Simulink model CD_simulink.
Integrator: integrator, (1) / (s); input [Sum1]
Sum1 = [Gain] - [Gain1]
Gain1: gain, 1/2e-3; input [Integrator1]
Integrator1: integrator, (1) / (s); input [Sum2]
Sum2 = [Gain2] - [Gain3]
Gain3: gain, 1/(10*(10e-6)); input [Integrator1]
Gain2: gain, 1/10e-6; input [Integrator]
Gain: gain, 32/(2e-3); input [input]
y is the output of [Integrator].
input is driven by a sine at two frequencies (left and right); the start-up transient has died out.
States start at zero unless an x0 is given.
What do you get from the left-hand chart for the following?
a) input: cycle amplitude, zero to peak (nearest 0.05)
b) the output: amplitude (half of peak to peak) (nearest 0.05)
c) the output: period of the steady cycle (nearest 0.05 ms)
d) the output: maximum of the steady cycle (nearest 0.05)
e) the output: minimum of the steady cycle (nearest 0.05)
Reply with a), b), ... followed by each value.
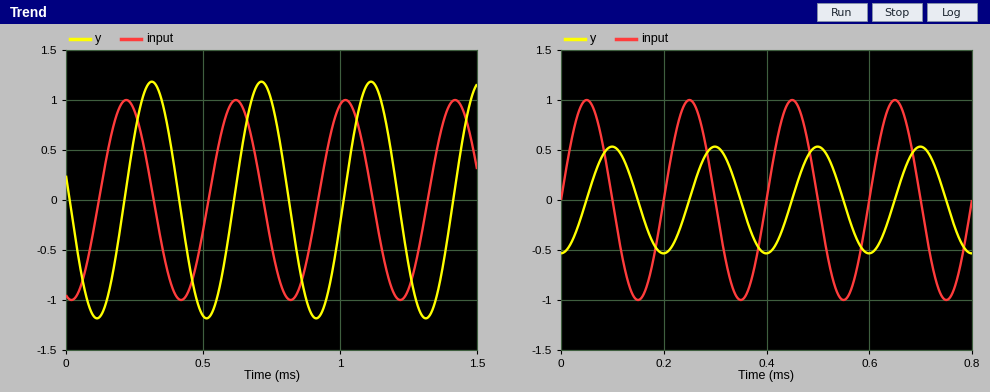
a) 1.00
b) 1.20
c) 0.40 ms
d) 1.20
e) -1.20
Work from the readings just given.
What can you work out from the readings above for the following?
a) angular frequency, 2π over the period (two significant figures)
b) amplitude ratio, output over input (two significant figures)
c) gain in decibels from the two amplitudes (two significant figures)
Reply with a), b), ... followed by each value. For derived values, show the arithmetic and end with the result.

a) 2π / 0.4 = 16 rad/ms
b) 1.2 / 1 = 1.2
c) 20 log10(1.2 / 1) = 1.6 dB
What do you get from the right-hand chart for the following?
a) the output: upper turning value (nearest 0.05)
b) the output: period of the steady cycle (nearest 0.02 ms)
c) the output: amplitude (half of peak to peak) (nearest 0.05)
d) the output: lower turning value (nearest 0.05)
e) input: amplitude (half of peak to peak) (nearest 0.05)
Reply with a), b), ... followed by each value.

a) 0.55
b) 0.20 ms
c) 0.55
d) -0.55
e) 1.00
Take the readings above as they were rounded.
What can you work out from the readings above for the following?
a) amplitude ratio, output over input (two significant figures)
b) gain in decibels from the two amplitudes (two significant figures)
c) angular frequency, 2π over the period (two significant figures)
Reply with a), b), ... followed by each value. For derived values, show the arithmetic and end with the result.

a) 0.55 / 1 = 0.55
b) 20 log10(0.55 / 1) = -5.2 dB
c) 2π / 0.2 = 31 rad/ms
